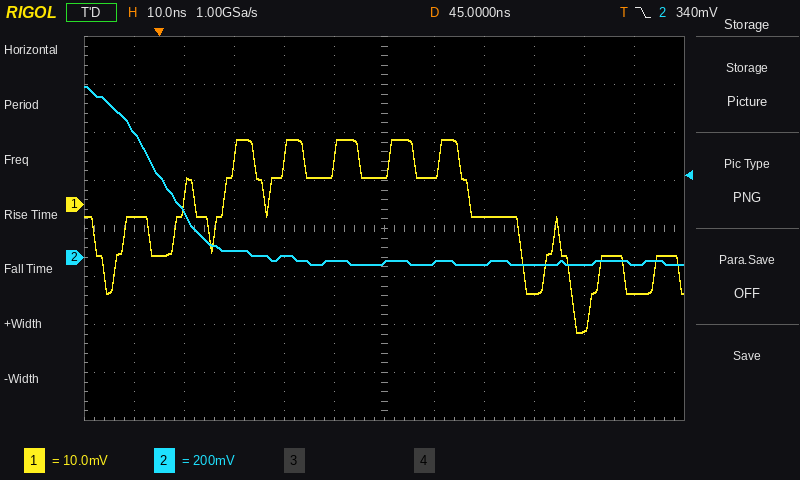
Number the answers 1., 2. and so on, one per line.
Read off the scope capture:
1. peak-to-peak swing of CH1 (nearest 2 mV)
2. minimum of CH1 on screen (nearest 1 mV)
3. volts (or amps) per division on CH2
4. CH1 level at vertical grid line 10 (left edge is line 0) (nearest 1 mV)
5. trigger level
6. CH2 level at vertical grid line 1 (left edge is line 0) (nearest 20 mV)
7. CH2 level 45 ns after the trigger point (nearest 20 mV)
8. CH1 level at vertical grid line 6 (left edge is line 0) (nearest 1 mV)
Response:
1. 40 mV
2. -27 mV
3. 200 mV
4. -26 mV
5. 340 mV
6. 520 mV
7. -20 mV
8. 6 mV
